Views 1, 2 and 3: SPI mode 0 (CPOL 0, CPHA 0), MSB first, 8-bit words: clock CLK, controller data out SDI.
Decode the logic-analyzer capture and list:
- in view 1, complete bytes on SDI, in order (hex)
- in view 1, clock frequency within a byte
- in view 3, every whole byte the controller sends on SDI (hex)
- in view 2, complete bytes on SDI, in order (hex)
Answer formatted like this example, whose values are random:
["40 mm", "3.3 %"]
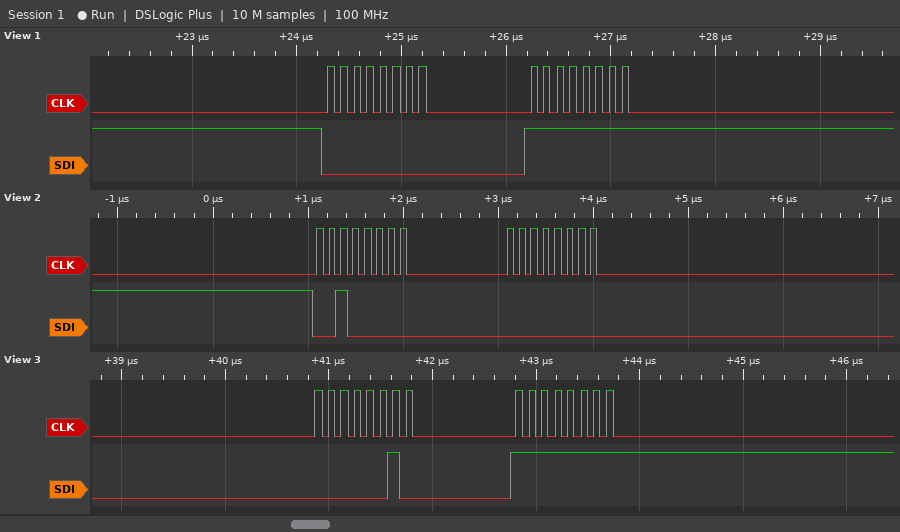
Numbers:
["00 FF", "8 MHz", "02 FF", "20 00"]
